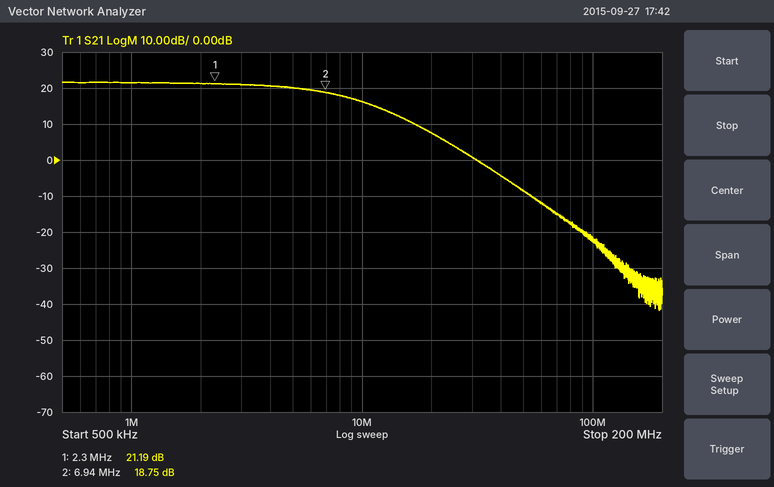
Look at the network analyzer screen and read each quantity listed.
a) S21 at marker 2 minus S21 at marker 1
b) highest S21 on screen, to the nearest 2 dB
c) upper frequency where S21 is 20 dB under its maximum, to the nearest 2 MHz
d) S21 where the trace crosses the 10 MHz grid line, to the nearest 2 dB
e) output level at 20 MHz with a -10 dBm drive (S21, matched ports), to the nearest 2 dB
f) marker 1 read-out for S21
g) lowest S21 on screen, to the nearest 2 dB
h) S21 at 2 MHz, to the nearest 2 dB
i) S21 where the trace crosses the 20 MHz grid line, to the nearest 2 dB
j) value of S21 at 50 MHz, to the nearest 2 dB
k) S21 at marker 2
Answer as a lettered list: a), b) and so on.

a) -2.44 dB
b) 22 dB
c) 28 MHz
d) 16 dB
e) -2 dBm
f) 21.19 dB
g) -42 dB
h) 22 dB
i) 8 dB
j) -8 dB
k) 18.75 dB
